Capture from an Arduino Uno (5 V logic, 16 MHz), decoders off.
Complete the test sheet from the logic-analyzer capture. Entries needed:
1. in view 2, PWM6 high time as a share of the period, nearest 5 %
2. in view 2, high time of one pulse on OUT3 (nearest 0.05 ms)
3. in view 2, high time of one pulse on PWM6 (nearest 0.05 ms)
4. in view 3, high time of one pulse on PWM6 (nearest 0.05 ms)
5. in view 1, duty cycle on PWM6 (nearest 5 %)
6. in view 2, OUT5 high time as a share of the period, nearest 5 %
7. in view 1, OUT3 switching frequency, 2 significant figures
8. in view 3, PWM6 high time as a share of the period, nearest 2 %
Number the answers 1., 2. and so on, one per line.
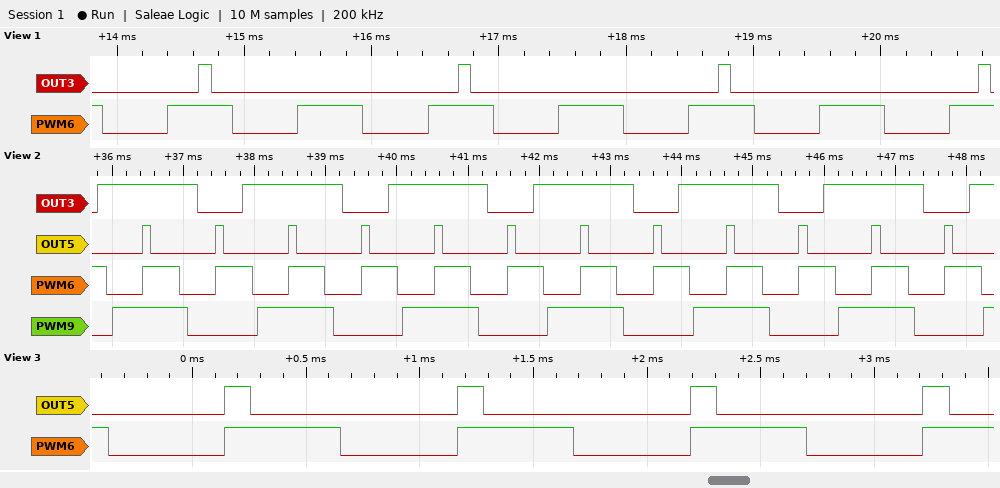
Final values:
1. 50 %
2. 1.40 ms
3. 0.50 ms
4. 0.50 ms
5. 50 %
6. 10 %
7. 490 Hz
8. 50 %
